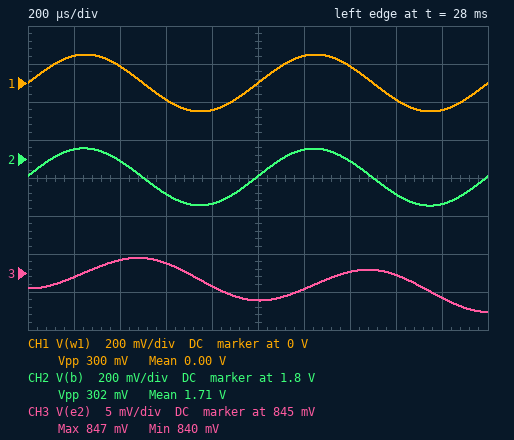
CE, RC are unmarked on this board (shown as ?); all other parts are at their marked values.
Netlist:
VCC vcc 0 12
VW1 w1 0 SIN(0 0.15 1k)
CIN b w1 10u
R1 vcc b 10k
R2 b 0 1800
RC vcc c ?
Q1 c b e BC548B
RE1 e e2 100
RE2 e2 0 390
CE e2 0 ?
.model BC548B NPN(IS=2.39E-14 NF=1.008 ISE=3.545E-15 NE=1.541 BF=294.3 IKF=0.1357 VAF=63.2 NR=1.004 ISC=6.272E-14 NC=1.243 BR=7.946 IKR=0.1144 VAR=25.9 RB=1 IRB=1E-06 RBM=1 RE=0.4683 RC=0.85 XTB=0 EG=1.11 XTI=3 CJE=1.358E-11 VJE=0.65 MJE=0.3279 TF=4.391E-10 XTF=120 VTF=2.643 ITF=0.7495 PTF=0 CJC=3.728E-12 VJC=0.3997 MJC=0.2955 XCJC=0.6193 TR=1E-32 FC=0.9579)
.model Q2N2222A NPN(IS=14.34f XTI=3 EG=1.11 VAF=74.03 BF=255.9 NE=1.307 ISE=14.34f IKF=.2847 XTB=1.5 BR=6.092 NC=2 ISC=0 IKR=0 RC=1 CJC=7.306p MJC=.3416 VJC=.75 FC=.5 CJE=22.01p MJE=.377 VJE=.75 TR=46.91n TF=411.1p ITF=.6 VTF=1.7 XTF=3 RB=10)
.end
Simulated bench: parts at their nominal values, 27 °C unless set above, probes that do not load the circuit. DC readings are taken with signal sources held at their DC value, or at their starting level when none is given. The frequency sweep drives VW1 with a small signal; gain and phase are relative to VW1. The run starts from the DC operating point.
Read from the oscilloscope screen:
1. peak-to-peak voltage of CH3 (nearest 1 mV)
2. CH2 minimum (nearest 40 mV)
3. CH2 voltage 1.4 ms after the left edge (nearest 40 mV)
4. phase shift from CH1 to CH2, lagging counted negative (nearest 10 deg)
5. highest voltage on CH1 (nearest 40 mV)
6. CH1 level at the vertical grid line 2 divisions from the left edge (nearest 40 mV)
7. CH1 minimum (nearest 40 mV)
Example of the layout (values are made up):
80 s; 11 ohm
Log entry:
7 mV; 1.56 V; 1.80 V; 0 deg; 160 mV; 80 mV; -160 mV
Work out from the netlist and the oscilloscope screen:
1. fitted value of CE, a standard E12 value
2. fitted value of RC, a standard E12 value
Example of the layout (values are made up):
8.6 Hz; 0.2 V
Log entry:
82 µF; 3.9 kΩ
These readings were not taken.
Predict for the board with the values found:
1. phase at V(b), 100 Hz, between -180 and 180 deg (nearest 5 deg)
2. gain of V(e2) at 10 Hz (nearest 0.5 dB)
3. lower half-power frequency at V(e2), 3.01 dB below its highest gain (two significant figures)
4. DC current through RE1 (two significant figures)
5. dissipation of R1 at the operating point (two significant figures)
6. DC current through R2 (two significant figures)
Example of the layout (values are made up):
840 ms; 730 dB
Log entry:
5 deg; -6.5 dB; 6.0 Hz; 2.4 mA; 10 mW; 1.0 mA
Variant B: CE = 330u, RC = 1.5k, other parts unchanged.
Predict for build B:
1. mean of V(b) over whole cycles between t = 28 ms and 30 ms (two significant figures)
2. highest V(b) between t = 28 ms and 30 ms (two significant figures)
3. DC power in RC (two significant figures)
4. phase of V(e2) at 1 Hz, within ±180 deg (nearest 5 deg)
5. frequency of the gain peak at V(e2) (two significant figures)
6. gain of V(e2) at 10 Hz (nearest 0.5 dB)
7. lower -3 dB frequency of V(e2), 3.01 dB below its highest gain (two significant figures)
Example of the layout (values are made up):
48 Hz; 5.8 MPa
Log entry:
1.8 V; 2.0 V; 8.3 mW; 75 deg; 7.6 Hz; -12.0 dB; 3.0 Hz
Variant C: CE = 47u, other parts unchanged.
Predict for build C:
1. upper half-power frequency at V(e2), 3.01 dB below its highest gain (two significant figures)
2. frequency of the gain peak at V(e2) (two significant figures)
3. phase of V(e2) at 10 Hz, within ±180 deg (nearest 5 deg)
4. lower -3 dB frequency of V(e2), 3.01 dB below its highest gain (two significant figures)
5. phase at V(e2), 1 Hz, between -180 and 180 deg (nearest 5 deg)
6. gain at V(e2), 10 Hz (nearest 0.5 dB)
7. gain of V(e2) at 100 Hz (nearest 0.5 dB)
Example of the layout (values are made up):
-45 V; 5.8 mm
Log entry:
57 Hz; 20 Hz; 30 deg; 7.2 Hz; 85 deg; -6.0 dB; -11.0 dB
